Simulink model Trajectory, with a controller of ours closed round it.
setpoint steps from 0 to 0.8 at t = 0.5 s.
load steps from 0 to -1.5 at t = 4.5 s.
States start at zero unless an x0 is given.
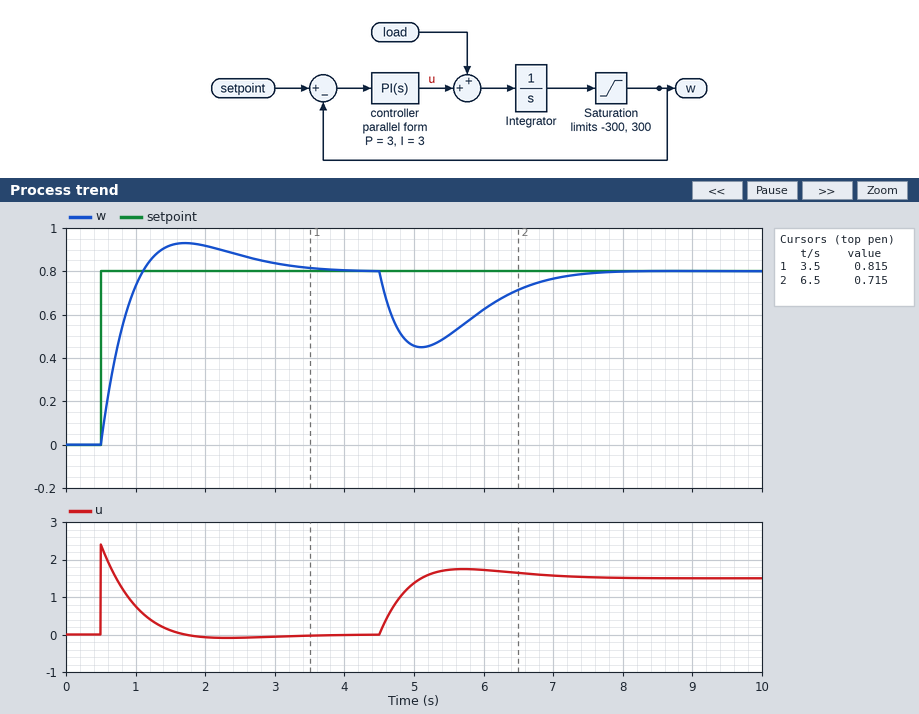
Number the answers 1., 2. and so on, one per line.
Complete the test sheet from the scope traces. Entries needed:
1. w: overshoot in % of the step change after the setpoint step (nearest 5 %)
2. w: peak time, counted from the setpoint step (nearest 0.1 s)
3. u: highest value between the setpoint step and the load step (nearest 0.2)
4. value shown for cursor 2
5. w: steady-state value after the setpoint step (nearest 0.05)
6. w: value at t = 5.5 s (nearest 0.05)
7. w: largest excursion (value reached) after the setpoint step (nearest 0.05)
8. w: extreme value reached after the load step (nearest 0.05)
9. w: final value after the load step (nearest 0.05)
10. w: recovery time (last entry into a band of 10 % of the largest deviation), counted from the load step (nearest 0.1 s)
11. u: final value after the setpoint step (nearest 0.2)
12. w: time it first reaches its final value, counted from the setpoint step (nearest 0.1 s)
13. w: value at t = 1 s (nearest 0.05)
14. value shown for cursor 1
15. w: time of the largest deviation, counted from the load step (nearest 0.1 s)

1. 15 %
2. 1.2 s
3. 2.4
4. 0.715
5. 0.80
6. 0.50
7. 0.95
8. 0.45
9. 0.80
10. 2.5 s
11. 0.0
12. 0.6 s
13. 0.75
14. 0.815
15. 0.6 s
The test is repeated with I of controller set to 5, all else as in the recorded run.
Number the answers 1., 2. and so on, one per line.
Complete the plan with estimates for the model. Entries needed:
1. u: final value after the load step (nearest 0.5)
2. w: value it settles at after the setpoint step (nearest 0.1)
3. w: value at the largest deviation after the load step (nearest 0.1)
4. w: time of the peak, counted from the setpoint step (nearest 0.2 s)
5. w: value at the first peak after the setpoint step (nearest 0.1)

1. 1.5
2. 0.8
3. 0.5
4. 1.0 s
5. 1.0
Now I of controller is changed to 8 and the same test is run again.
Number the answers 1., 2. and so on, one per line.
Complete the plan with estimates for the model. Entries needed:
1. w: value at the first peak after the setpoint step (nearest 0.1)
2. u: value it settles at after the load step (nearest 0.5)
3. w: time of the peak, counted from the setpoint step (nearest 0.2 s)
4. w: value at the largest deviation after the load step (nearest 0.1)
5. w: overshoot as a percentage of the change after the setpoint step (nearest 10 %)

1. 1.0
2. 1.5
3. 0.8 s
4. 0.5
5. 30 %
